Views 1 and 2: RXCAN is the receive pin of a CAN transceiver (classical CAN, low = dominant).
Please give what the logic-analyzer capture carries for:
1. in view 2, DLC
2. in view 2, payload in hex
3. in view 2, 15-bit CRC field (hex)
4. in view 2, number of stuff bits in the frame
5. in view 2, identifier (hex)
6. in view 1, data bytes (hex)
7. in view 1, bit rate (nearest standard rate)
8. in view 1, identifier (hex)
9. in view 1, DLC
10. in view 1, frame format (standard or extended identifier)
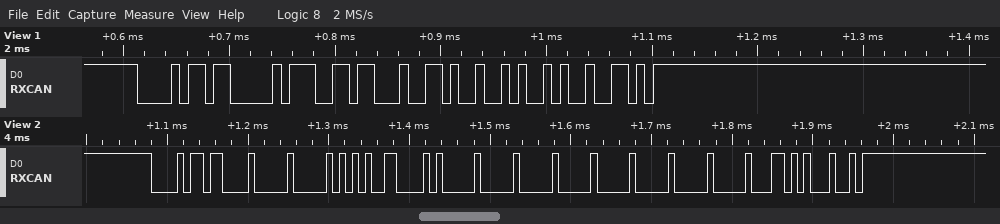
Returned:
8
00 A9 85 00 00 00 00 00
0x0D44
10
0x0B6
9B 13 49
125 kbit/s
0x0B6
3
standard
